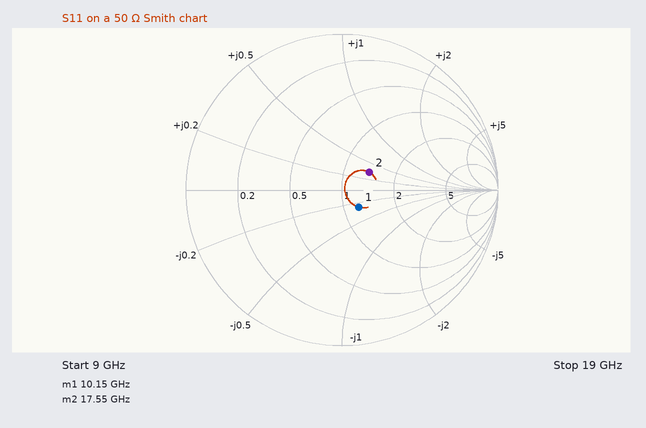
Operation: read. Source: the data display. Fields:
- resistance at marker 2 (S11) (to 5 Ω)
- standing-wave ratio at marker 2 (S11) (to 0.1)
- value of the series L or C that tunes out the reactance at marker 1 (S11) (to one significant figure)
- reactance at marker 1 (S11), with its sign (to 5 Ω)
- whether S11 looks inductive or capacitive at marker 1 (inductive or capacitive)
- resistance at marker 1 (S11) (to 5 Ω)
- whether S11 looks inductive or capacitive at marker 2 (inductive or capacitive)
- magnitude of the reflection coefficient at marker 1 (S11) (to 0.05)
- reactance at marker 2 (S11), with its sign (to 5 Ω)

70 Ω
1.5
200 pH
-15 Ω
capacitive
60 Ω
inductive
0.15
+15 Ω
